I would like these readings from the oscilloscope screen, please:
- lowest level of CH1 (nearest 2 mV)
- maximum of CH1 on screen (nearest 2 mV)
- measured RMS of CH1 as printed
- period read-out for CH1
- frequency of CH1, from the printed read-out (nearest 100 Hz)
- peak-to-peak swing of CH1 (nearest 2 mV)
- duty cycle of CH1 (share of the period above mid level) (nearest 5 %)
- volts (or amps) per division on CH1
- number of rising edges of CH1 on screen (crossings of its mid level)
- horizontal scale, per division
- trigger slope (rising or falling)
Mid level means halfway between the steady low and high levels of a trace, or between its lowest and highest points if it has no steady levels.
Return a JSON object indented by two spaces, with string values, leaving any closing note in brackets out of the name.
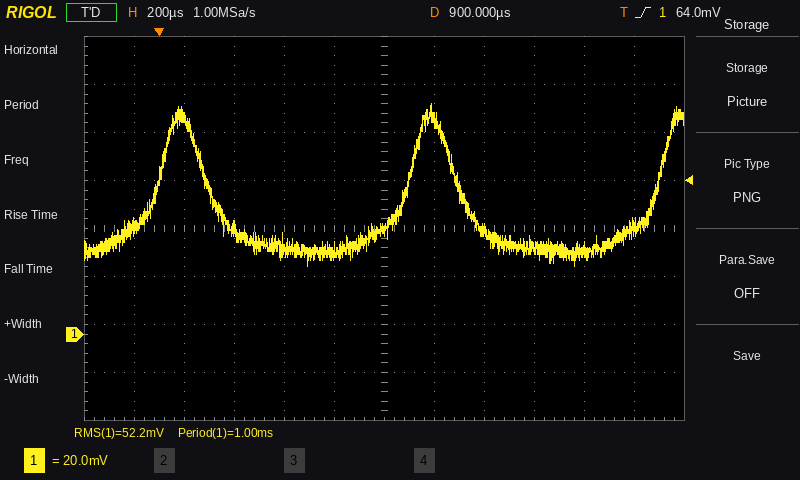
{
  "lowest level of CH1": "28 mV",
  "maximum of CH1 on screen": "96 mV",
  "measured RMS of CH1 as printed": "52.2 mV",
  "period read-out for CH1": "1.00 ms",
  "frequency of CH1, from the printed read-out": "1.0 kHz",
  "peak-to-peak swing of CH1": "68 mV",
  "duty cycle of CH1 (share of the period above mid level)": "20 %",
  "volts (or amps) per division on CH1": "20 mV",
  "number of rising edges of CH1 on screen": "3",
  "horizontal scale, per division": "200 µs",
  "trigger slope": "rising"
}
